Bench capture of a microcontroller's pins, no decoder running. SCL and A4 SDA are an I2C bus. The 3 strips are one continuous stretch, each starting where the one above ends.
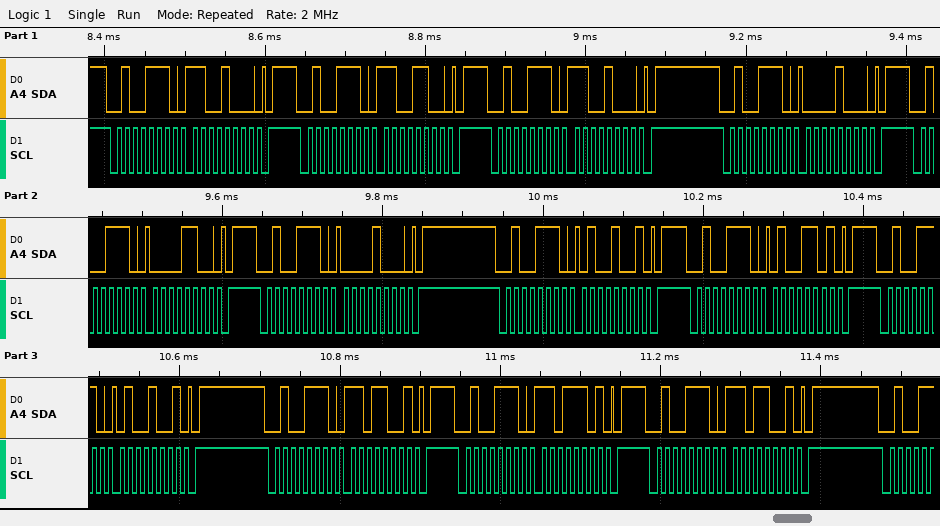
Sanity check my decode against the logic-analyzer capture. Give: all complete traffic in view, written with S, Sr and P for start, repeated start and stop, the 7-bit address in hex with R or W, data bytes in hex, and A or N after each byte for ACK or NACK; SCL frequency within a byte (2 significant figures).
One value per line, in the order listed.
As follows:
S 27W A C8 A P S 27W A CC A P S 27W A C8 A P S 27W A 08 A P S 27W A 0C A P S 27W A 08 A P S 27W A 49 A P S 27W A 4D A P S 27W A 49 A P S 27W A D9 A P S 27W A DD A P S 27W A D9 A P
100 kHz
